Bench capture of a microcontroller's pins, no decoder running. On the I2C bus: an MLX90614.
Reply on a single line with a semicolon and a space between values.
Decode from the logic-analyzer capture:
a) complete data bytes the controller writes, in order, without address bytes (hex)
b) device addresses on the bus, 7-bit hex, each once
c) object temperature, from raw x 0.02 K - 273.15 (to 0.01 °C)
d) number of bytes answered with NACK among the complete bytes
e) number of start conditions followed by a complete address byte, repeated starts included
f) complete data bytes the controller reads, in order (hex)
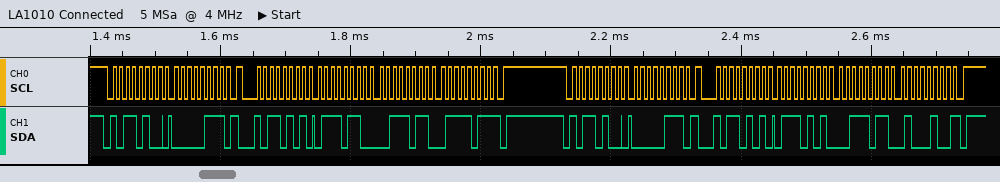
07 07; 0x5A; 31.29 °C; 2; 4; 76 3B 7B 75 3B 44
